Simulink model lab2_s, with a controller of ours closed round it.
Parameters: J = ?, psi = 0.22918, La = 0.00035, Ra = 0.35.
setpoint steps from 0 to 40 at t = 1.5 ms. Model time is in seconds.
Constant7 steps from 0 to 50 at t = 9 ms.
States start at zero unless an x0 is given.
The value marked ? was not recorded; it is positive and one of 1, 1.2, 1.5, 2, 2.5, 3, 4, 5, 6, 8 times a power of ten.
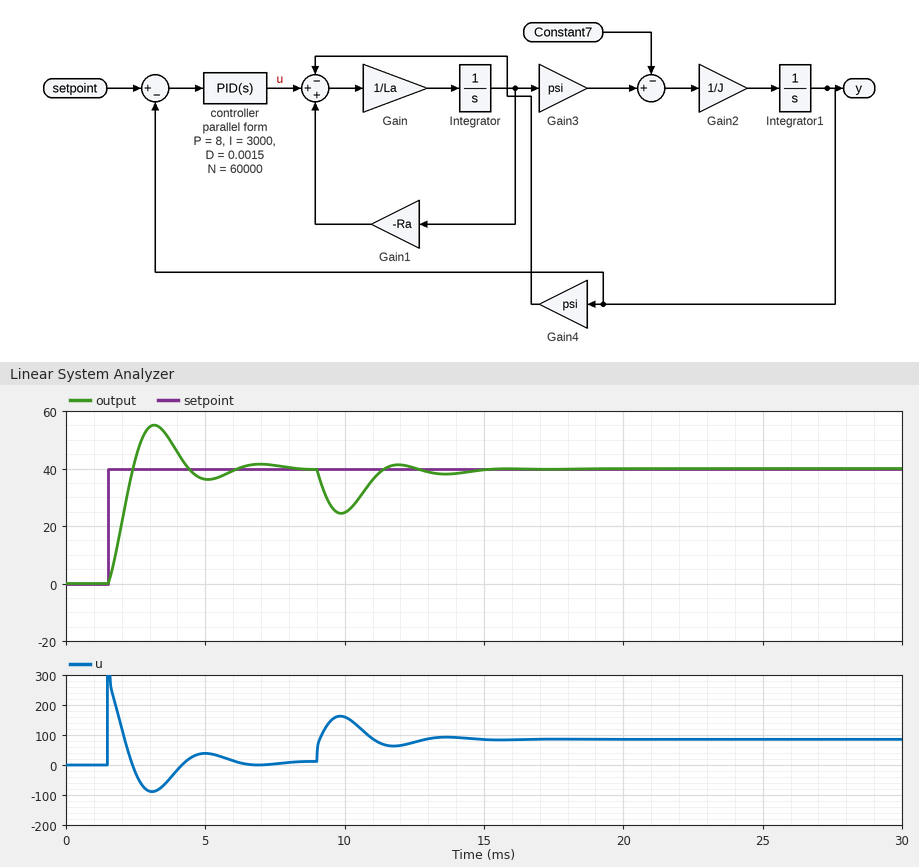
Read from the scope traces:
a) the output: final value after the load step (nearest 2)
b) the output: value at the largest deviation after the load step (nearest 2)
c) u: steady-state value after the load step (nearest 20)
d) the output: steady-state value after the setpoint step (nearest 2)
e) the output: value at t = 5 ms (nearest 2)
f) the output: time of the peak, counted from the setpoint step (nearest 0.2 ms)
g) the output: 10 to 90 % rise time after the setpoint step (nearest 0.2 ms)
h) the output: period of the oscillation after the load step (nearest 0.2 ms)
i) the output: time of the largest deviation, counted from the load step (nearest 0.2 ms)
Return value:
40
24
80
40
36
1.6 ms
0.6 ms
3.8 ms
0.8 ms
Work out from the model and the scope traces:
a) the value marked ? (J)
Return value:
0.0015
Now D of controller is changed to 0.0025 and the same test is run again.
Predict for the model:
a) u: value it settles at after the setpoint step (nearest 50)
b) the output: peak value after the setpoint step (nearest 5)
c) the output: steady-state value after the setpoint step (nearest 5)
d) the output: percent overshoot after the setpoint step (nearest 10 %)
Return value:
0
50
40
30 %
